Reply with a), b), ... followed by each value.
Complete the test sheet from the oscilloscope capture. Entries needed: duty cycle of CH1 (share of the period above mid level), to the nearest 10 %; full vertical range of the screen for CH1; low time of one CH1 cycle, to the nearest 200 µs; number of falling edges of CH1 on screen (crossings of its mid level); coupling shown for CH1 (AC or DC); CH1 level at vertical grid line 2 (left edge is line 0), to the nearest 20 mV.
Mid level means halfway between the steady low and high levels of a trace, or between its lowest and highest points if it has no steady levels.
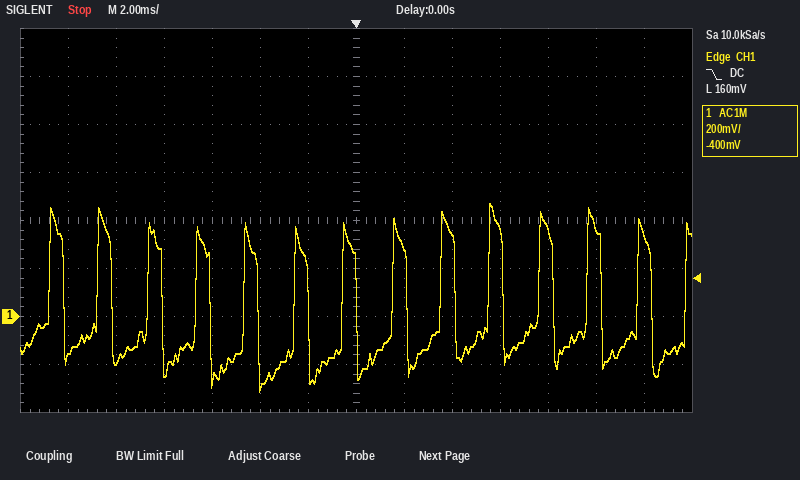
a) 30 %
b) 1.6 V
c) 1.4 ms
d) 13
e) AC
f) -200 mV
